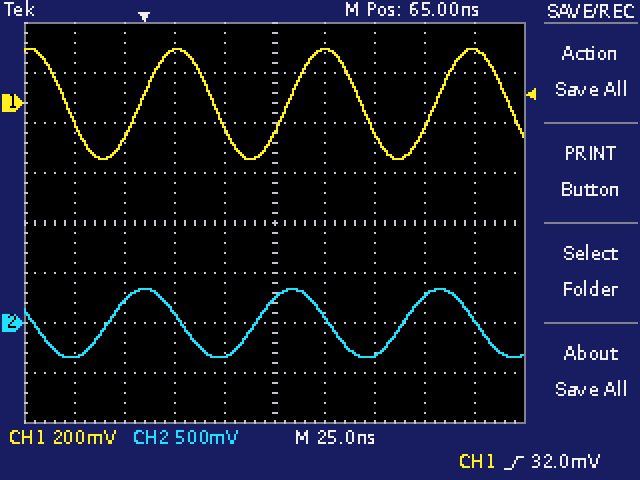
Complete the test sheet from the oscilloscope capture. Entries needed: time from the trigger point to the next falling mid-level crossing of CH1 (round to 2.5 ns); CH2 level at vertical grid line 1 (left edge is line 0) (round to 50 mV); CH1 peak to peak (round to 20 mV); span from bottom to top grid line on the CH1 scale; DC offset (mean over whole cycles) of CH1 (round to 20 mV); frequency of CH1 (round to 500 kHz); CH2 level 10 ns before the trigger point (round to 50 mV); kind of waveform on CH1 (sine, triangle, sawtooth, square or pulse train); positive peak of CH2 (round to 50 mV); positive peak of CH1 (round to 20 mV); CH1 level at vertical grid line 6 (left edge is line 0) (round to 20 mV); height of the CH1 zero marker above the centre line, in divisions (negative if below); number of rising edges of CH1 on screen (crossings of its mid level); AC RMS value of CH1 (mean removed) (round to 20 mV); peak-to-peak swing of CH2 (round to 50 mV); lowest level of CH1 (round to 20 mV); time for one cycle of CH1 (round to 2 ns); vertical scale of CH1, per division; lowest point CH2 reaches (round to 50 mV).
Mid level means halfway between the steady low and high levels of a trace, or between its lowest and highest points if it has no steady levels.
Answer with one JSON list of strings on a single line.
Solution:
["35.0 ns", "-350 mV", "440 mV", "1.6 V", "0 mV", "13.5 MHz", "200 mV", "sine", "350 mV", "220 mV", "220 mV", "+2.4 div", "3", "160 mV", "700 mV", "-220 mV", "74 ns", "200 mV", "-350 mV"]
